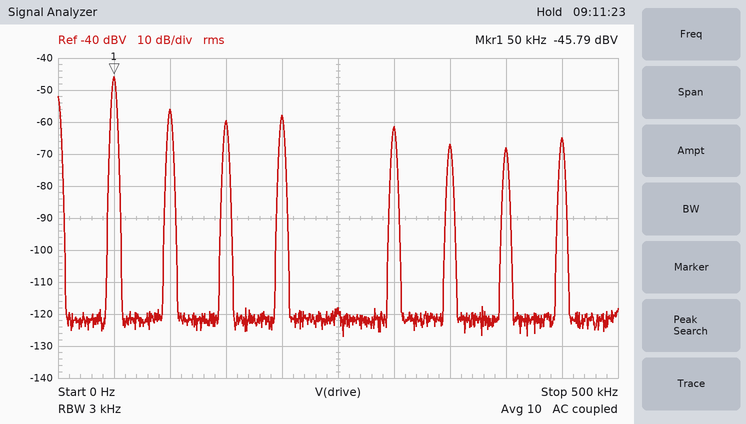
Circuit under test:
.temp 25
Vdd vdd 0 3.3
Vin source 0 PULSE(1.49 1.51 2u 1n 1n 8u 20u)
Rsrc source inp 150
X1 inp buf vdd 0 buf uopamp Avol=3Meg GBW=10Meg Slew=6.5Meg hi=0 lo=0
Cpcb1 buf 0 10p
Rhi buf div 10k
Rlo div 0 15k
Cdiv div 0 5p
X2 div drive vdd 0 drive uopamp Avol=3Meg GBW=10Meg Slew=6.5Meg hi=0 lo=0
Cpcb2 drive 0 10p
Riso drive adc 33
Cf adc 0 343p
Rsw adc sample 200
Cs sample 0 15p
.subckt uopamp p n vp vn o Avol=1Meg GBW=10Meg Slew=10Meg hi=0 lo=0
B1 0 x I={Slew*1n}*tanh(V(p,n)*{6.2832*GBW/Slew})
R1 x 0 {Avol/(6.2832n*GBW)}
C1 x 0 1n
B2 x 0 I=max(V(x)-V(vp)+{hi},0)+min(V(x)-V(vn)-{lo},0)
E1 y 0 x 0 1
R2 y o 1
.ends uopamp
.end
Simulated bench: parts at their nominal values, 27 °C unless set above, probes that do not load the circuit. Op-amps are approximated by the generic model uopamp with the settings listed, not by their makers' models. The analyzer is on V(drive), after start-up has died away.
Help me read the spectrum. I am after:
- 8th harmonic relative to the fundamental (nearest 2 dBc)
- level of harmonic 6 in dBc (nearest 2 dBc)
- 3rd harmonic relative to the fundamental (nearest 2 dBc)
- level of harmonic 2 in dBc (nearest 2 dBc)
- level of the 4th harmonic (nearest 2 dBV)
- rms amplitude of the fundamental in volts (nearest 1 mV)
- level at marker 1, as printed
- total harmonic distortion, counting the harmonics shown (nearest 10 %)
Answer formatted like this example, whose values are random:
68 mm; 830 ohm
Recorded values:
-22 dBc; -16 dBc; -14 dBc; -10 dBc; -58 dBV; 5 mV; -45.79 dBV; 50 %
